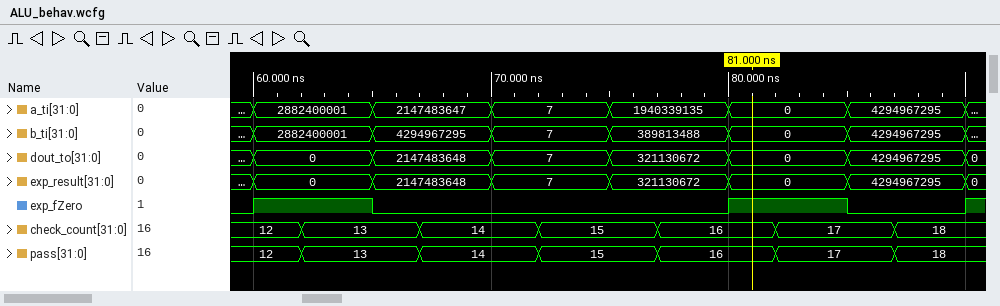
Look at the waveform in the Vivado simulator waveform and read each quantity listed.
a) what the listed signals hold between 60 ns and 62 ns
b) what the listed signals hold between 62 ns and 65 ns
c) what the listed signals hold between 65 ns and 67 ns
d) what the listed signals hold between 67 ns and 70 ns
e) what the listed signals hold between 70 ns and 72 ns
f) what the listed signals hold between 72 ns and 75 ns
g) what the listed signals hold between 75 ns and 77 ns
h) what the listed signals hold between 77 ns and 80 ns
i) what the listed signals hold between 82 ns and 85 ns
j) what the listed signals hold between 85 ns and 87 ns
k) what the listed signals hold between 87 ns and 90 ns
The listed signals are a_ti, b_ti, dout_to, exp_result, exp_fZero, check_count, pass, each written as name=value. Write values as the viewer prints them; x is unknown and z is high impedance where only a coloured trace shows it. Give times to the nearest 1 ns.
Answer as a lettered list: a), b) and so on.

a) a_ti=2882400001, b_ti=2882400001, dout_to=0, exp_result=0, exp_fZero=1, check_count=12, pass=12
b) a_ti=2882400001, b_ti=2882400001, dout_to=0, exp_result=0, exp_fZero=1, check_count=13, pass=13
c) a_ti=2147483647, b_ti=4294967295, dout_to=2147483648, exp_result=2147483648, exp_fZero=0, check_count=13, pass=13
d) a_ti=2147483647, b_ti=4294967295, dout_to=2147483648, exp_result=2147483648, exp_fZero=0, check_count=14, pass=14
e) a_ti=7, b_ti=7, dout_to=7, exp_result=7, exp_fZero=0, check_count=14, pass=14
f) a_ti=7, b_ti=7, dout_to=7, exp_result=7, exp_fZero=0, check_count=15, pass=15
g) a_ti=1940339135, b_ti=389813488, dout_to=321130672, exp_result=321130672, exp_fZero=0, check_count=15, pass=15
h) a_ti=1940339135, b_ti=389813488, dout_to=321130672, exp_result=321130672, exp_fZero=0, check_count=16, pass=16
i) a_ti=0, b_ti=0, dout_to=0, exp_result=0, exp_fZero=1, check_count=17, pass=17
j) a_ti=4294967295, b_ti=4294967295, dout_to=4294967295, exp_result=4294967295, exp_fZero=0, check_count=17, pass=17
k) a_ti=4294967295, b_ti=4294967295, dout_to=4294967295, exp_result=4294967295, exp_fZero=0, check_count=18, pass=18
